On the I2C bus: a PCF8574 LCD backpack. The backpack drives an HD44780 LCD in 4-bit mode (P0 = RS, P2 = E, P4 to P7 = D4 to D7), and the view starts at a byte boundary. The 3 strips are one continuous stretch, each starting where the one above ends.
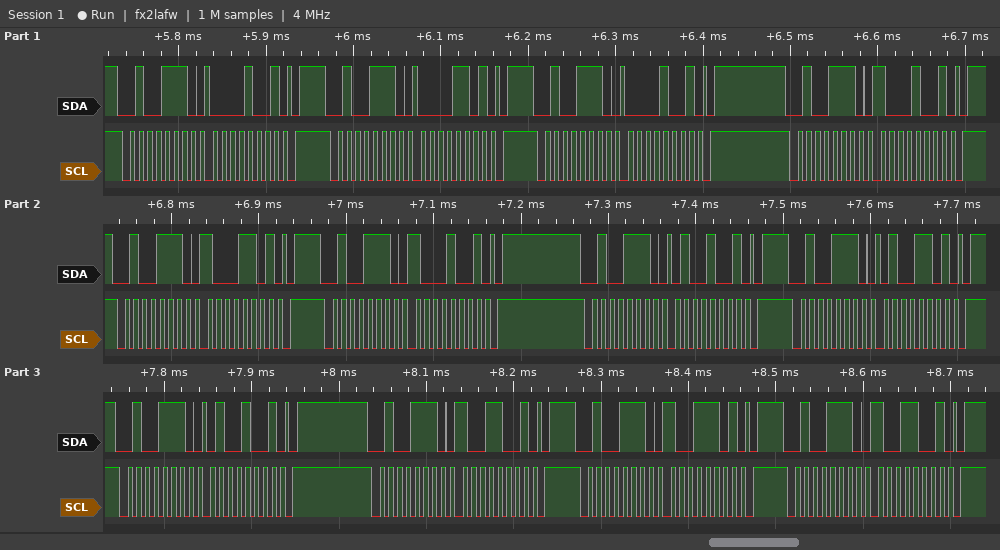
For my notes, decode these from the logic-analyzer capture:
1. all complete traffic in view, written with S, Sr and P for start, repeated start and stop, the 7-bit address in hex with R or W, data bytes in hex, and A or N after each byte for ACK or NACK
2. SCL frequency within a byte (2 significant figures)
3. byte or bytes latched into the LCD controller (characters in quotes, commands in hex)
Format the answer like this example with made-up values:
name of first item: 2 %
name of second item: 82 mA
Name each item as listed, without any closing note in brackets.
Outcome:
all complete traffic in view, written with S, Sr and P for start, repeated start and stop, the 7-bit address in hex with R or W, data bytes in hex, and A or N after each byte for ACK or NACK: S 27W A 09 A P S 27W A 0D A P S 27W A 09 A P S 27W A 89 A P S 27W A 8D A P S 27W A 89 A P S 27W A 49 A P S 27W A 4D A P S 27W A 49 A P S 27W A 99 A P S 27W A 9D A P S 27W A 99 A P
SCL frequency within a byte: 100 kHz
byte or bytes latched into the LCD controller: data 0x08 'I'
